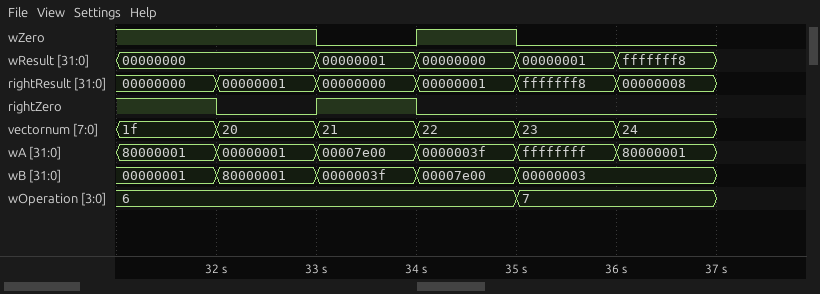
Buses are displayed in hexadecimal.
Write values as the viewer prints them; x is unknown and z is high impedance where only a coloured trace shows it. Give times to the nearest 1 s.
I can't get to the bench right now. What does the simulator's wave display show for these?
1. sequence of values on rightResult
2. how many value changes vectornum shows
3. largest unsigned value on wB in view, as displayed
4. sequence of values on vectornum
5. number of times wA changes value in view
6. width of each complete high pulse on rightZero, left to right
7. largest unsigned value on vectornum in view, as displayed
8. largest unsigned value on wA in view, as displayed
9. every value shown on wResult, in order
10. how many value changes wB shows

00000000, 00000001, 00000000, 00000001, fffffff8, 00000008
5
80000001
1f, 20, 21, 22, 23, 24
5
1 s
24
ffffffff
00000000, 00000001, 00000000, 00000001, fffffff8
4
